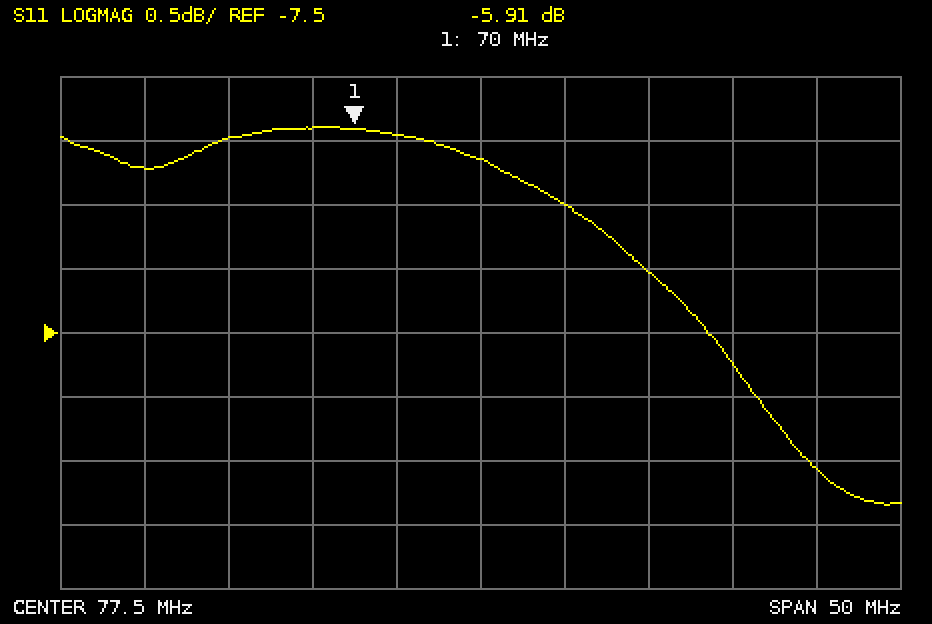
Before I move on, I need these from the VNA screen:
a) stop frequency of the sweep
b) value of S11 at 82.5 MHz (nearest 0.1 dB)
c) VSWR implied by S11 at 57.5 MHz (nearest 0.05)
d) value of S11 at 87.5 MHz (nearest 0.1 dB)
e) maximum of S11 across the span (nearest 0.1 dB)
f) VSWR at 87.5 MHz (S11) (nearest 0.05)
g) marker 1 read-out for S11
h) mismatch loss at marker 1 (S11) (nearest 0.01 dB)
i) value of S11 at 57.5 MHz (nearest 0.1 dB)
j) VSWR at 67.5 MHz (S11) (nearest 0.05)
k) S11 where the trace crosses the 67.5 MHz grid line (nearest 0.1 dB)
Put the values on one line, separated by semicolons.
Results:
102.5 MHz; -6.5 dB; 2.90; -7.0 dB; -5.9 dB; 2.60; -5.91 dB; 1.29 dB; -6.2 dB; 3.05; -5.9 dB
